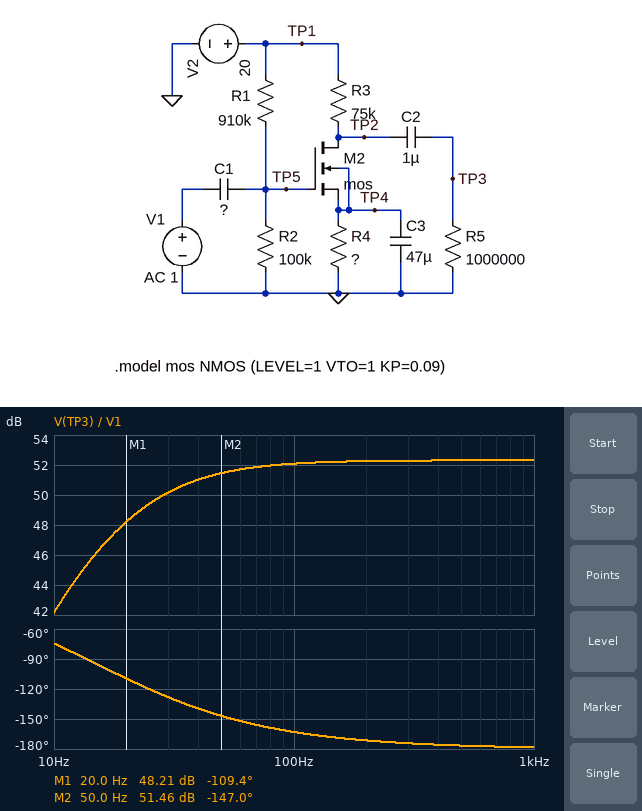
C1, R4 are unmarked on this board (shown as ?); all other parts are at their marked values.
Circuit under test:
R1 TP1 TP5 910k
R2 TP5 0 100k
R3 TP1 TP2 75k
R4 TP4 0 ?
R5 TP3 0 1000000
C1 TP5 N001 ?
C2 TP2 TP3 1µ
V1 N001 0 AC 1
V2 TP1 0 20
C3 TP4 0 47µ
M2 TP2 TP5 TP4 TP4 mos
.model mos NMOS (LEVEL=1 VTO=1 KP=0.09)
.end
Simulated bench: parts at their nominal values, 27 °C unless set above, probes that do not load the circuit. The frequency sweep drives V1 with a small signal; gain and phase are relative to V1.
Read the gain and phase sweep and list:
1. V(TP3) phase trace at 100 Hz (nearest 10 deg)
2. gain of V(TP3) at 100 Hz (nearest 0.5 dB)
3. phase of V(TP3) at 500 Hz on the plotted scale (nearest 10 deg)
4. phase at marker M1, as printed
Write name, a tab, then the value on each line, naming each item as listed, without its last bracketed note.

V(TP3) phase trace at 100 Hz	-160 deg
gain of V(TP3) at 100 Hz	52.0 dB
phase of V(TP3) at 500 Hz on the plotted scale	-180 deg
phase at marker M1, as printed	-109.4 deg
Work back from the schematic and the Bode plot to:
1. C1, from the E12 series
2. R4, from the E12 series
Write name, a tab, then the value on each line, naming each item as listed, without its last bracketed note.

C1, from the E12 series	180 nF
R4, from the E12 series	4.7 kΩ
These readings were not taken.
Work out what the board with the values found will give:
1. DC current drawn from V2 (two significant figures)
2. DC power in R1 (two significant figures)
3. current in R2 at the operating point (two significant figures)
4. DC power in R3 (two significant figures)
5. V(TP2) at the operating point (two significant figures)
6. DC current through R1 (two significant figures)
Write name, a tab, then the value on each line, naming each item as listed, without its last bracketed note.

DC current drawn from V2	210 µA
DC power in R1	360 µW
current in R2 at the operating point	20 µA
DC power in R3	2.8 mW
V(TP2) at the operating point	5.4 V
DC current through R1	20 µA
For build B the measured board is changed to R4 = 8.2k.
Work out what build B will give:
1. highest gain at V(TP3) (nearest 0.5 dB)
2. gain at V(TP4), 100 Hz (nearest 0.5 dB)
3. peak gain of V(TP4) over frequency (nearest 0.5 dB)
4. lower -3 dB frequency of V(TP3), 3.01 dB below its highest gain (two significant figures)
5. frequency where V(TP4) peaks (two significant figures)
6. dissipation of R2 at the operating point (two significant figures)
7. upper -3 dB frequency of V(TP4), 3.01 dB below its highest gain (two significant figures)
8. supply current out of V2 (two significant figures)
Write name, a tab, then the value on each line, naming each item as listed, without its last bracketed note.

highest gain at V(TP3)	50.0 dB
gain at V(TP4), 100 Hz	-16.5 dB
peak gain of V(TP4) over frequency	-4.5 dB
lower -3 dB frequency of V(TP3), 3.01 dB below its highest gain	20 Hz
frequency where V(TP4) peaks	12 Hz
dissipation of R2 at the operating point	39 µW
upper -3 dB frequency of V(TP4), 3.01 dB below its highest gain	31 Hz
supply current out of V2	130 µA
